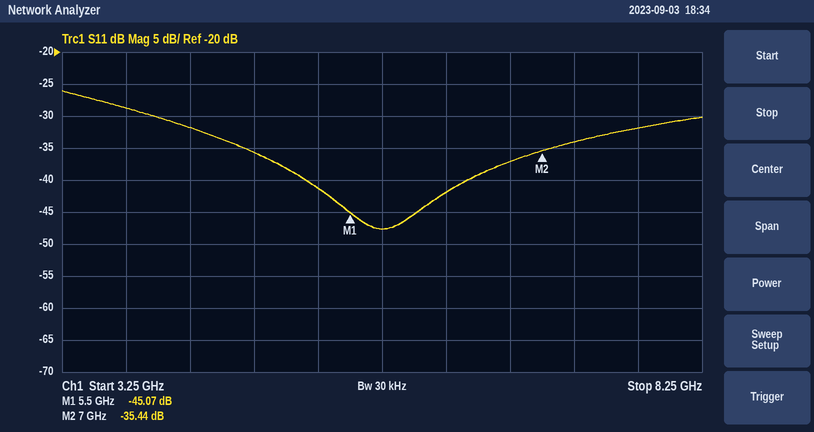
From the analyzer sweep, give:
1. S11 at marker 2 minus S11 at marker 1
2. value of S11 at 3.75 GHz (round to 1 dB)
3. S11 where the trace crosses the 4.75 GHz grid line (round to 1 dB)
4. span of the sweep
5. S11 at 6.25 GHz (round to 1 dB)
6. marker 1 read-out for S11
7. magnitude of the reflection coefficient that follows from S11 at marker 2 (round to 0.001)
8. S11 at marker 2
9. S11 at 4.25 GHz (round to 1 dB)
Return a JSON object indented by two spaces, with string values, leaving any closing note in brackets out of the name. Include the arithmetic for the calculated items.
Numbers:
{
  "S11 at marker 2 minus S11 at marker 1": "-35.44 − (-45.07) = 9.63 dB",
  "value of S11 at 3.75 GHz": "-29 dB",
  "S11 where the trace crosses the 4.75 GHz grid line": "-36 dB",
  "span of the sweep": "5 GHz",
  "S11 at 6.25 GHz": "-42 dB",
  "marker 1 read-out for S11": "-45.07 dB",
  "magnitude of the reflection coefficient that follows from S11 at marker 2": "10^(-35.44/20) ≈ 0.017",
  "S11 at marker 2": "-35.44 dB",
  "S11 at 4.25 GHz": "-32 dB"
}
